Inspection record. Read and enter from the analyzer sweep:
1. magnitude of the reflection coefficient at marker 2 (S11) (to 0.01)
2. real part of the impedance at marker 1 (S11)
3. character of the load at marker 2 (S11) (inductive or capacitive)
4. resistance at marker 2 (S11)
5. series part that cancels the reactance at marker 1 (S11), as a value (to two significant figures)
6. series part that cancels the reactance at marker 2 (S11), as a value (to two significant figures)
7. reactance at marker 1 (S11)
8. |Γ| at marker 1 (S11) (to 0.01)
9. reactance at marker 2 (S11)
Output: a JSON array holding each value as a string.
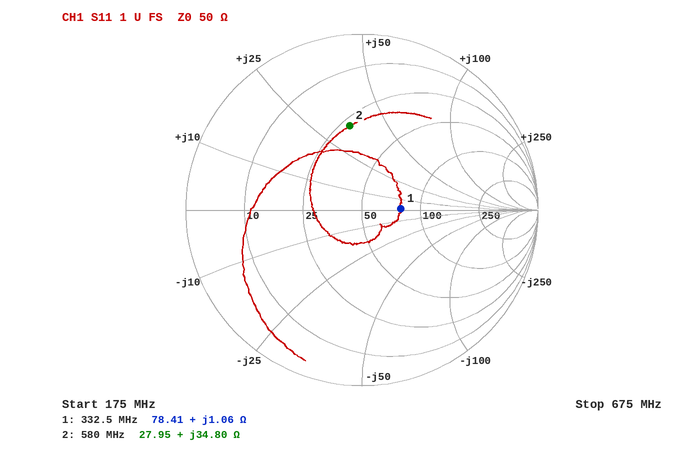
["0.48", "78.41 Ω", "inductive", "27.95 Ω", "450 pF", "7.9 pF", "+1.06 Ω", "0.22", "+34.80 Ω"]
